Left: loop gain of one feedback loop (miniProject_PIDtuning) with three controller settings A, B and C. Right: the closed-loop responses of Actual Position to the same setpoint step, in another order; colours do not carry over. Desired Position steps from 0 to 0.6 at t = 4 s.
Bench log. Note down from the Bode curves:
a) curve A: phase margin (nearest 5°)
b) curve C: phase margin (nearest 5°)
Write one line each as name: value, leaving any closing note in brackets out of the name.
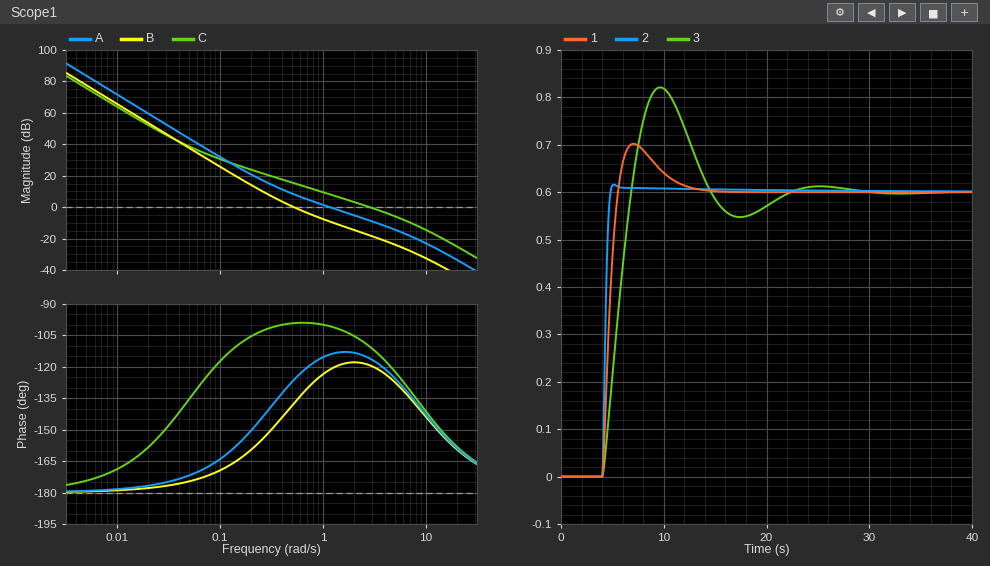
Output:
curve A: phase margin: 65°
curve C: phase margin: 70°
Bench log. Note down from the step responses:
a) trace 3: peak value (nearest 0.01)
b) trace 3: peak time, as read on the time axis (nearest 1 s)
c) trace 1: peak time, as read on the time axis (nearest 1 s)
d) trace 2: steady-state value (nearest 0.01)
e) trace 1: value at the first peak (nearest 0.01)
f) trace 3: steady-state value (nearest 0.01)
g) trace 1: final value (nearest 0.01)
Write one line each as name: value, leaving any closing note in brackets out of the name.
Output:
trace 3: peak value: 0.82
trace 3: peak time, as read on the time axis: 10 s
trace 1: peak time, as read on the time axis: 7 s
trace 2: steady-state value: 0.60
trace 1: value at the first peak: 0.70
trace 3: steady-state value: 0.60
trace 1: final value: 0.60
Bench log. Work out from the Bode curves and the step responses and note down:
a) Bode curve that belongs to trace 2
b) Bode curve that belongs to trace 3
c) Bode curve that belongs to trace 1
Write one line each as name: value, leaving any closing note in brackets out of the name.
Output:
Bode curve that belongs to trace 2: C
Bode curve that belongs to trace 3: B
Bode curve that belongs to trace 1: A
